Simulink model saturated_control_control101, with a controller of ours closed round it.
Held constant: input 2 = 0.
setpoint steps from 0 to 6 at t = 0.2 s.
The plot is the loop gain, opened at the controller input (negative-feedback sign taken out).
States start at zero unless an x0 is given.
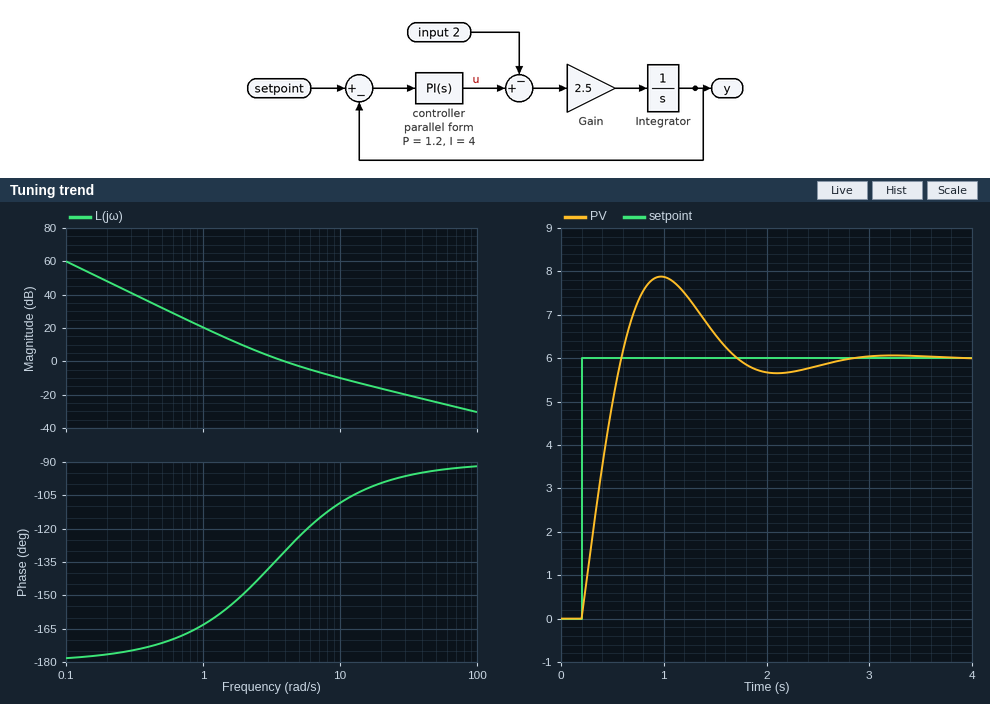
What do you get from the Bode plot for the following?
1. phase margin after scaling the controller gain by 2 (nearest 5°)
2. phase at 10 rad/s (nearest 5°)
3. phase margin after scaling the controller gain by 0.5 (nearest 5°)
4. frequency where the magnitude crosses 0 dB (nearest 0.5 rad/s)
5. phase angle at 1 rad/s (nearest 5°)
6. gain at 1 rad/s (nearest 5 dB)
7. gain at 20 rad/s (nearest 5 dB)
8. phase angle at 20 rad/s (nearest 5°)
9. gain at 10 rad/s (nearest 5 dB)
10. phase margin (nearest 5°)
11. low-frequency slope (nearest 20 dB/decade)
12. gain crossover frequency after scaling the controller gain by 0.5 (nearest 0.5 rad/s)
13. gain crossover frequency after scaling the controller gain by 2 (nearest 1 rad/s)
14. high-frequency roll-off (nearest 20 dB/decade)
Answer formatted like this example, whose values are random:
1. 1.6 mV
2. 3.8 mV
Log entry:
1. 65°
2. -110°
3. 35°
4. 4.0 rad/s
5. -165°
6. 20 dB
7. -15 dB
8. -100°
9. -10 dB
10. 50°
11. -40 dB/decade
12. 2.5 rad/s
13. 7 rad/s
14. -20 dB/decade
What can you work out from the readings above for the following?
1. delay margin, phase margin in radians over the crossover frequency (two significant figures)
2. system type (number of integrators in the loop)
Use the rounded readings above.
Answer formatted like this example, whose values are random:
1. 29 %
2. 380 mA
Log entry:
1. 0.22 s
2. 2
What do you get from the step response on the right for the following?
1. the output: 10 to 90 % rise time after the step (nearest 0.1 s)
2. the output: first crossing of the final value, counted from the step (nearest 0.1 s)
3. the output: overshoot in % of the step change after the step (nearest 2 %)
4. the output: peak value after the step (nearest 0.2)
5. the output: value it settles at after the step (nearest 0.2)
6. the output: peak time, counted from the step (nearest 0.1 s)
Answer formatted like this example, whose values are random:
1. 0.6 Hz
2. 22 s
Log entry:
1. 0.3 s
2. 0.4 s
3. 32 %
4. 7.8
5. 6.0
6. 0.8 s
